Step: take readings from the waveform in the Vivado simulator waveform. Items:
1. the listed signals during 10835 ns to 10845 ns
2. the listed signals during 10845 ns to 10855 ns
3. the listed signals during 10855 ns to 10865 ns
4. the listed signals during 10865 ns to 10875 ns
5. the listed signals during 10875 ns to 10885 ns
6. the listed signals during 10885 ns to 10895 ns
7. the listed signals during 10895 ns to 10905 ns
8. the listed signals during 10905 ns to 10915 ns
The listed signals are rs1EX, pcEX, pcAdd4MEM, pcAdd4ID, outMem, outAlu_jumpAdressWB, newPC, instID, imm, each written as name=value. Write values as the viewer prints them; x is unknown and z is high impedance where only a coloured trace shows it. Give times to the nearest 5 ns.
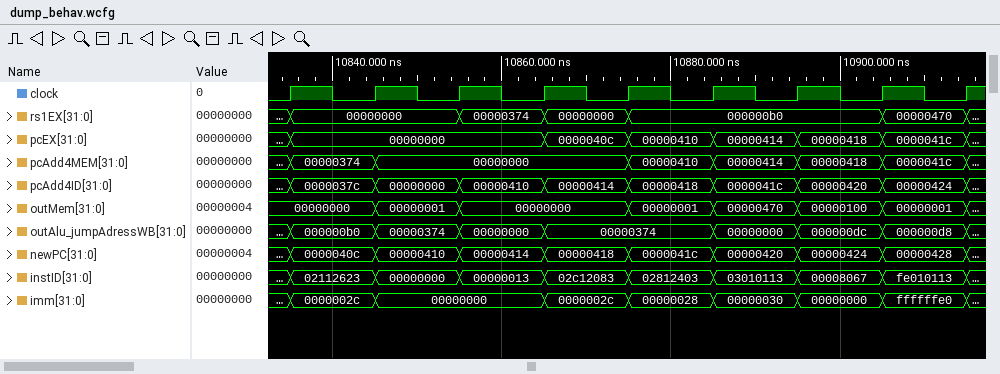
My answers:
rs1EX=00000000, pcEX=00000000, pcAdd4MEM=00000374, pcAdd4ID=0000037c, outMem=00000000, outAlu_jumpAdressWB=000000b0, newPC=0000040c, instID=02112623, imm=0000002c
rs1EX=00000000, pcEX=00000000, pcAdd4MEM=00000000, pcAdd4ID=00000000, outMem=00000001, outAlu_jumpAdressWB=00000374, newPC=00000410, instID=00000000, imm=00000000
rs1EX=00000374, pcEX=00000000, pcAdd4MEM=00000000, pcAdd4ID=00000410, outMem=00000000, outAlu_jumpAdressWB=00000000, newPC=00000414, instID=00000013, imm=00000000
rs1EX=00000000, pcEX=0000040c, pcAdd4MEM=00000000, pcAdd4ID=00000414, outMem=00000000, outAlu_jumpAdressWB=00000374, newPC=00000418, instID=02c12083, imm=0000002c
rs1EX=000000b0, pcEX=00000410, pcAdd4MEM=00000410, pcAdd4ID=00000418, outMem=00000001, outAlu_jumpAdressWB=00000374, newPC=0000041c, instID=02812403, imm=00000028
rs1EX=000000b0, pcEX=00000414, pcAdd4MEM=00000414, pcAdd4ID=0000041c, outMem=00000470, outAlu_jumpAdressWB=00000000, newPC=00000420, instID=03010113, imm=00000030
rs1EX=000000b0, pcEX=00000418, pcAdd4MEM=00000418, pcAdd4ID=00000420, outMem=00000100, outAlu_jumpAdressWB=000000dc, newPC=00000424, instID=00008067, imm=00000000
rs1EX=00000470, pcEX=0000041c, pcAdd4MEM=0000041c, pcAdd4ID=00000424, outMem=00000001, outAlu_jumpAdressWB=000000d8, newPC=00000428, instID=fe010113, imm=ffffffe0
